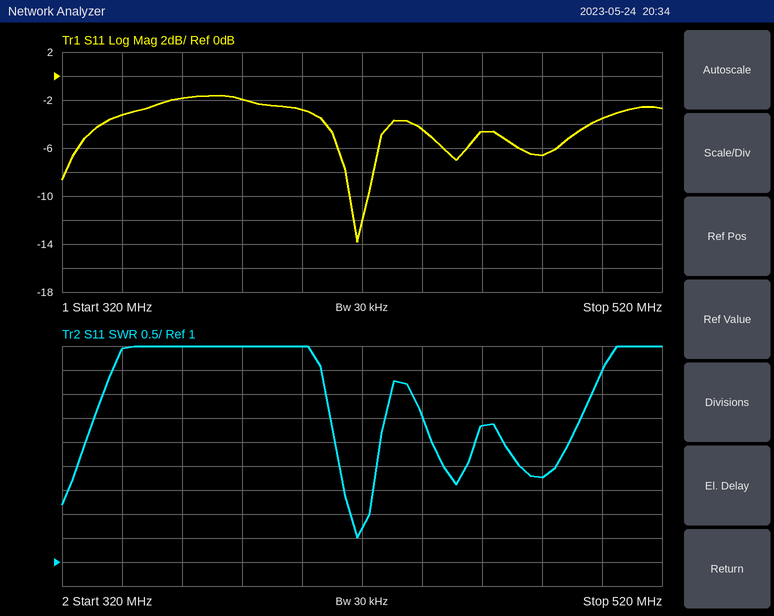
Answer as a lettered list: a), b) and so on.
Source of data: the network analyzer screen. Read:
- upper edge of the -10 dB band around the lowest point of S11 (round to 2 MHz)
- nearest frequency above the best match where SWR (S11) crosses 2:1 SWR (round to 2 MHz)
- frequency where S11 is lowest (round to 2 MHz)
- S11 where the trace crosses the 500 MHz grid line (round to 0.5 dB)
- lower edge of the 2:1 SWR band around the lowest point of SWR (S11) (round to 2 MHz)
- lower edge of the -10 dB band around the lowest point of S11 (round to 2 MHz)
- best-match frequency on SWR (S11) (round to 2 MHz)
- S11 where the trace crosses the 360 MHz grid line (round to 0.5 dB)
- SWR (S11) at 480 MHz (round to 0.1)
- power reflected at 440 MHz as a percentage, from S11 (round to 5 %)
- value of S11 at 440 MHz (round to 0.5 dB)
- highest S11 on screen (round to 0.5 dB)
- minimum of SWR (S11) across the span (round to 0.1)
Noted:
a) 422 MHz
b) 422 MHz
c) 418 MHz
d) -3.5 dB
e) 416 MHz
f) 416 MHz
g) 418 MHz
h) -2.0 dB
i) 2.8
j) 35 %
k) -4.5 dB
l) -1.5 dB
m) 1.5
